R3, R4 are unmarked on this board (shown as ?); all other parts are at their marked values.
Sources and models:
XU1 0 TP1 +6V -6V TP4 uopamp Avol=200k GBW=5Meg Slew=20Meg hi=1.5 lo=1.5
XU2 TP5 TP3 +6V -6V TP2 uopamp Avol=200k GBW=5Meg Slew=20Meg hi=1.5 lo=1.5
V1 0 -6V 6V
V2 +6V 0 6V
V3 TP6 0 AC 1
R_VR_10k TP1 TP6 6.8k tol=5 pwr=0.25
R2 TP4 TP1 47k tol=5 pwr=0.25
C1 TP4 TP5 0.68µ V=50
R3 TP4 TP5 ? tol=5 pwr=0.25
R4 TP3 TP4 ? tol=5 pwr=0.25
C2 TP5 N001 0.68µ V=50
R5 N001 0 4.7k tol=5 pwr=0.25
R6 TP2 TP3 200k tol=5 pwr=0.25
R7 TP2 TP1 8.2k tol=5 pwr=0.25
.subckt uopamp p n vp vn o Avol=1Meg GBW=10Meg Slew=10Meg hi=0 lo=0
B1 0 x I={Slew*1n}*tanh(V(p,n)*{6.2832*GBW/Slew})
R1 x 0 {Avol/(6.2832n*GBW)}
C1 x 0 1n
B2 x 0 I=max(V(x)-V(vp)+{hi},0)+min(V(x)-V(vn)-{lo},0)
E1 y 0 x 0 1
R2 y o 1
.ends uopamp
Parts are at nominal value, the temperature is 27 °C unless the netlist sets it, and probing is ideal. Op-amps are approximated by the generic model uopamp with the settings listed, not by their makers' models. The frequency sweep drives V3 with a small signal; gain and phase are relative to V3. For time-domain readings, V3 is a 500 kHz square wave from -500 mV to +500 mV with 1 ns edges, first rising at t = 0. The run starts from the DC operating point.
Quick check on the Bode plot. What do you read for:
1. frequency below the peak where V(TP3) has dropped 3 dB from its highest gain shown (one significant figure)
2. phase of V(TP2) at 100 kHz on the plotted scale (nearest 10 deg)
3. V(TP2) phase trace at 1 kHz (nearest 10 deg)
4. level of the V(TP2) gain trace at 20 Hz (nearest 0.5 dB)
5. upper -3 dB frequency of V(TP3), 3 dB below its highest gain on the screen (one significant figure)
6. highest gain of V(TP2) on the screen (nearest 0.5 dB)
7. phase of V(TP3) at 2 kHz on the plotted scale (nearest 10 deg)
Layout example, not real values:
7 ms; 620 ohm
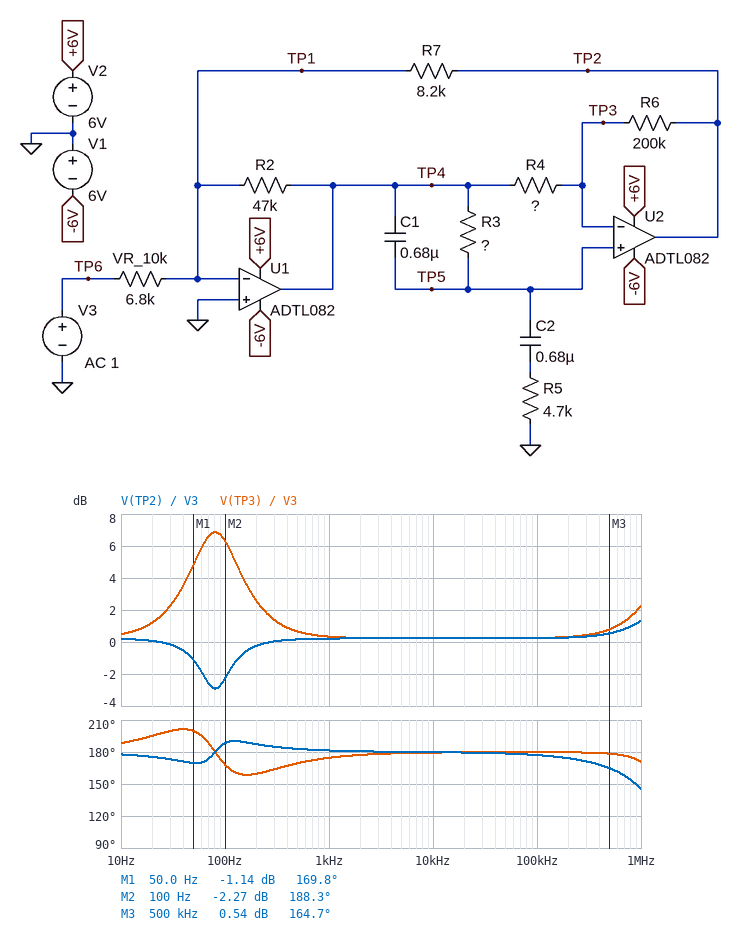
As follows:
40 Hz; 180 deg; 180 deg; 0 dB; 200 Hz; 1.5 dB; 180 deg
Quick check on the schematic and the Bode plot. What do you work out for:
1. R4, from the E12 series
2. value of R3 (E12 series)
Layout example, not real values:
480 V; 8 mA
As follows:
82 kΩ; 1.8 kΩ
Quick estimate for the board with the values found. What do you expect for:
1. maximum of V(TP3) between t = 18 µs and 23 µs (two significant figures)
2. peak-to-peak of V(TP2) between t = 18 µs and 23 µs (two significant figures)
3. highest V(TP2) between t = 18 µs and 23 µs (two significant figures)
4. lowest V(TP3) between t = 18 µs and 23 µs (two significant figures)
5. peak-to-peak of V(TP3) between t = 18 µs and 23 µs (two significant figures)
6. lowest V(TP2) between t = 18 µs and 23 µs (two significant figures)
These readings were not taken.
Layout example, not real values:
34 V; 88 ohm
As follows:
800 mV; 1.4 V; 690 mV; -820 mV; 1.6 V; -690 mV
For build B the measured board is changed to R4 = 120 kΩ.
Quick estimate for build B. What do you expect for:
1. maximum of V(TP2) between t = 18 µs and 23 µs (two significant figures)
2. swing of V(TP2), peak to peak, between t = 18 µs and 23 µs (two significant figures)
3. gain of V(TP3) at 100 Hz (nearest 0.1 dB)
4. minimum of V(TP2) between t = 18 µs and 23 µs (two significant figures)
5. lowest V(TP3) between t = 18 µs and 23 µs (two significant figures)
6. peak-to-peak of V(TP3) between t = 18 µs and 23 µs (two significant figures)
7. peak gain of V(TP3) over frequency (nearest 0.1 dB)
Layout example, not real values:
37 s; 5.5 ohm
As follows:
660 mV; 1.3 V; 3.8 dB; -660 mV; -720 mV; 1.4 V; 4.0 dB
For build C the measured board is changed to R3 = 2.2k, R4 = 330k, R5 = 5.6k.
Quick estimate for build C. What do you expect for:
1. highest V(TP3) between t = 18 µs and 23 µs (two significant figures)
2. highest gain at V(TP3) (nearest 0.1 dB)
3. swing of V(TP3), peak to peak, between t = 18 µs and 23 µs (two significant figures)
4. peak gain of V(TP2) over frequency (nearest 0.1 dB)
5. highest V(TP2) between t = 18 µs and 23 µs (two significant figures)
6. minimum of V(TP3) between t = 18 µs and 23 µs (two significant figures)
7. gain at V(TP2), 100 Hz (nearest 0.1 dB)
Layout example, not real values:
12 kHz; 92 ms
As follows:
600 mV; 1.2 dB; 1.2 V; 0.4 dB; 590 mV; -600 mV; -0.3 dB
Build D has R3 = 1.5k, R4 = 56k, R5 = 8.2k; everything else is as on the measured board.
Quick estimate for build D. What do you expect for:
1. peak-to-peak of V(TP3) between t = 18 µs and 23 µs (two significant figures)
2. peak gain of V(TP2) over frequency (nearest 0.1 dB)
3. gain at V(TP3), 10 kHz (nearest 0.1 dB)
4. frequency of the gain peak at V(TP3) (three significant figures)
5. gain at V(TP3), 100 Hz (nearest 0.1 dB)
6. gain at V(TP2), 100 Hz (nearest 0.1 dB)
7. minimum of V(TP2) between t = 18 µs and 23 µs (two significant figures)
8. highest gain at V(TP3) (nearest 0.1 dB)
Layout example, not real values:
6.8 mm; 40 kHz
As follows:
1.9 V; 2.2 dB; 0.2 dB; 66.7 Hz; 4.6 dB; -1.1 dB; -720 mV; 5.4 dB
